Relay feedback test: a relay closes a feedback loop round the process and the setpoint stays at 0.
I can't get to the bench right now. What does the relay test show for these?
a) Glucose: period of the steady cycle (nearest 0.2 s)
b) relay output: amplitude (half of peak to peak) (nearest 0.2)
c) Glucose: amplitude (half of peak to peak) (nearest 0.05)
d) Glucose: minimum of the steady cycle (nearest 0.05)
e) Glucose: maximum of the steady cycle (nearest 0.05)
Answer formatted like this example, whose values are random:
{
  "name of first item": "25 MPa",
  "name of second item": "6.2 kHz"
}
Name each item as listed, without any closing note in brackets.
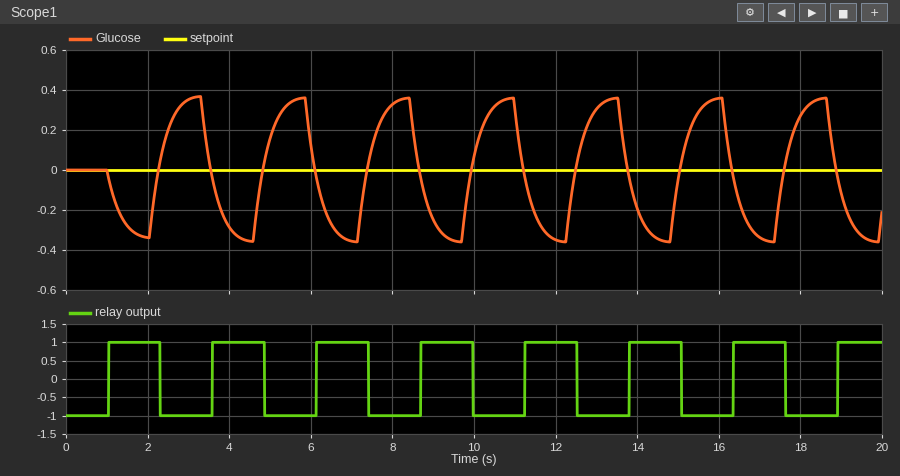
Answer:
{
  "Glucose: period of the steady cycle": "2.6 s",
  "relay output: amplitude (half of peak to peak)": "1.0",
  "Glucose: amplitude (half of peak to peak)": "0.35",
  "Glucose: minimum of the steady cycle": "-0.35",
  "Glucose: maximum of the steady cycle": "0.35"
}
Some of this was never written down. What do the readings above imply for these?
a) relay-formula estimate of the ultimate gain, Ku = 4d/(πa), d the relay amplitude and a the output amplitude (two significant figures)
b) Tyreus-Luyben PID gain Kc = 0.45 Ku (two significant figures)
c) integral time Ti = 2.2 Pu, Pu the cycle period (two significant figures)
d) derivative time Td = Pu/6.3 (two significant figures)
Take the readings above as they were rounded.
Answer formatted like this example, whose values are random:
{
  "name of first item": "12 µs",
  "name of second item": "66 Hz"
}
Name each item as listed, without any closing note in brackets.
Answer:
{
  "relay-formula estimate of the ultimate gain, Ku = 4d/(πa), d the relay amplitude and a the output amplitude": "3.6",
  "Tyreus-Luyben PID gain Kc = 0.45 Ku": "1.6",
  "integral time Ti = 2.2 Pu, Pu the cycle period": "5.7 s",
  "derivative time Td = Pu/6.3": "0.41 s"
}
